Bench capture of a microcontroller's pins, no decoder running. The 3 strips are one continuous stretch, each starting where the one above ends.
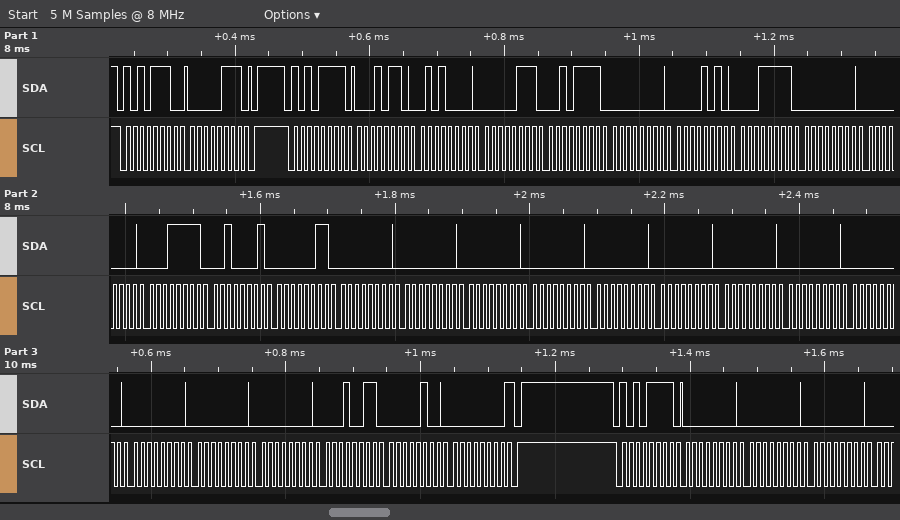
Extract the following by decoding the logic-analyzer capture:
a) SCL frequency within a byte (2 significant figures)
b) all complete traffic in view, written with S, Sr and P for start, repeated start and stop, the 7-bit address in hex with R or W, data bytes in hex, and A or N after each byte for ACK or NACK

100 kHz
S 57W A 07 A P S 57R A 16 A 50 A 07 A 2F A 00 A 0A A 1F A 00 A 00 A 1F A 21 A 03 A 00 A 00 A 00 A 00 A 00 A 00 A 00 A 00 A 00 A 00 A 00 A 00 A 13 A 04 A 00 N P S 57R A 00 A 00 A 00 A
